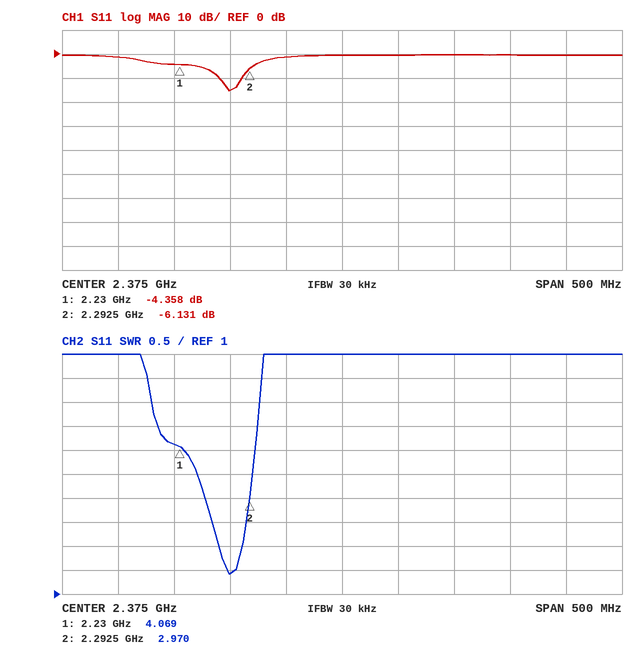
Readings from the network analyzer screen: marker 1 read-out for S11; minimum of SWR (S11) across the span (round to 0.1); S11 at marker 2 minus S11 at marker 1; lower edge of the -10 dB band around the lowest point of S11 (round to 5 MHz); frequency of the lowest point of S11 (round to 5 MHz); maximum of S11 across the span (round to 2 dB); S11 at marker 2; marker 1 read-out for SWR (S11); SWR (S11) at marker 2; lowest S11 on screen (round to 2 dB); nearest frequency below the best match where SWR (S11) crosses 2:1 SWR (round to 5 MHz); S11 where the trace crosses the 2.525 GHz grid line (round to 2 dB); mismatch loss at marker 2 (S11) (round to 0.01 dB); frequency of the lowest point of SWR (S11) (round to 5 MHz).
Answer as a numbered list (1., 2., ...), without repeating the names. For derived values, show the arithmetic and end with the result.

1. -4.358 dB
2. 1.4
3. -6.131 − (-4.358) = -1.773 dB
4. 2.265 GHz
5. 2.275 GHz
6. 0 dB
7. -6.131 dB
8. 4.069
9. 2.970
10. -16 dB
11. 2.265 GHz
12. 0 dB
13. −10 log10(1 − 10^(-6.131/10)) ≈ 1.21 dB
14. 2.275 GHz
